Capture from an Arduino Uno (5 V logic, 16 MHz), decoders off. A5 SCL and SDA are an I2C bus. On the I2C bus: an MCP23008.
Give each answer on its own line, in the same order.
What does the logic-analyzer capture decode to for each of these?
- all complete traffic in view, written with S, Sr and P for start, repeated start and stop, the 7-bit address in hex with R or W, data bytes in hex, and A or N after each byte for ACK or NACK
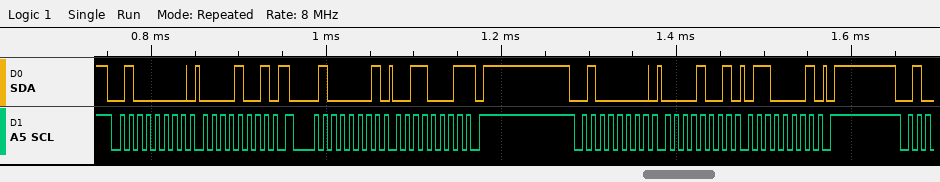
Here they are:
S 20W A 09 A Sr 20R A 31 N P S 20W A 09 A 61 A P
